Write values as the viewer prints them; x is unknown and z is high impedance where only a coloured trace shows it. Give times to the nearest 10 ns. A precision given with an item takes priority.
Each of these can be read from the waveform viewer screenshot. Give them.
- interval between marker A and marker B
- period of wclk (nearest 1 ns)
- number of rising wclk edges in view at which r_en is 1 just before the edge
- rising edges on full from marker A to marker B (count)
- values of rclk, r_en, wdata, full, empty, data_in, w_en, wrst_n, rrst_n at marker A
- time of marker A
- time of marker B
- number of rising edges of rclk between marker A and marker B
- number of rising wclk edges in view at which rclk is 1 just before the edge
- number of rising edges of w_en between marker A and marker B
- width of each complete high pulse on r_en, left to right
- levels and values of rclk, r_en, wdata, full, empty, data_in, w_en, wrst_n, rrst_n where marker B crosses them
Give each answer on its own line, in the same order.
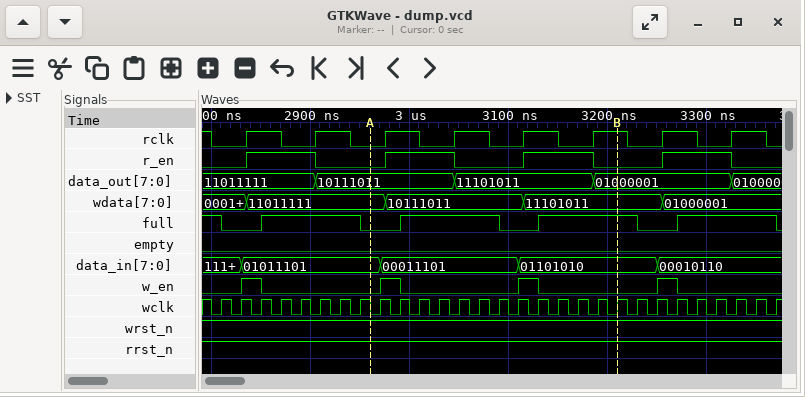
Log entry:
250 ns
20 ns
12
2
rclk=0, r_en=0, wdata=11011111, full=0, empty=0, data_in=01011101, w_en=0, wrst_n=1, rrst_n=1
2960 ns
3210 ns
4
16
2
70 ns, 70 ns, 70 ns, 70 ns
rclk=1, r_en=0, wdata=11101011, full=1, empty=0, data_in=01101010, w_en=0, wrst_n=1, rrst_n=1
